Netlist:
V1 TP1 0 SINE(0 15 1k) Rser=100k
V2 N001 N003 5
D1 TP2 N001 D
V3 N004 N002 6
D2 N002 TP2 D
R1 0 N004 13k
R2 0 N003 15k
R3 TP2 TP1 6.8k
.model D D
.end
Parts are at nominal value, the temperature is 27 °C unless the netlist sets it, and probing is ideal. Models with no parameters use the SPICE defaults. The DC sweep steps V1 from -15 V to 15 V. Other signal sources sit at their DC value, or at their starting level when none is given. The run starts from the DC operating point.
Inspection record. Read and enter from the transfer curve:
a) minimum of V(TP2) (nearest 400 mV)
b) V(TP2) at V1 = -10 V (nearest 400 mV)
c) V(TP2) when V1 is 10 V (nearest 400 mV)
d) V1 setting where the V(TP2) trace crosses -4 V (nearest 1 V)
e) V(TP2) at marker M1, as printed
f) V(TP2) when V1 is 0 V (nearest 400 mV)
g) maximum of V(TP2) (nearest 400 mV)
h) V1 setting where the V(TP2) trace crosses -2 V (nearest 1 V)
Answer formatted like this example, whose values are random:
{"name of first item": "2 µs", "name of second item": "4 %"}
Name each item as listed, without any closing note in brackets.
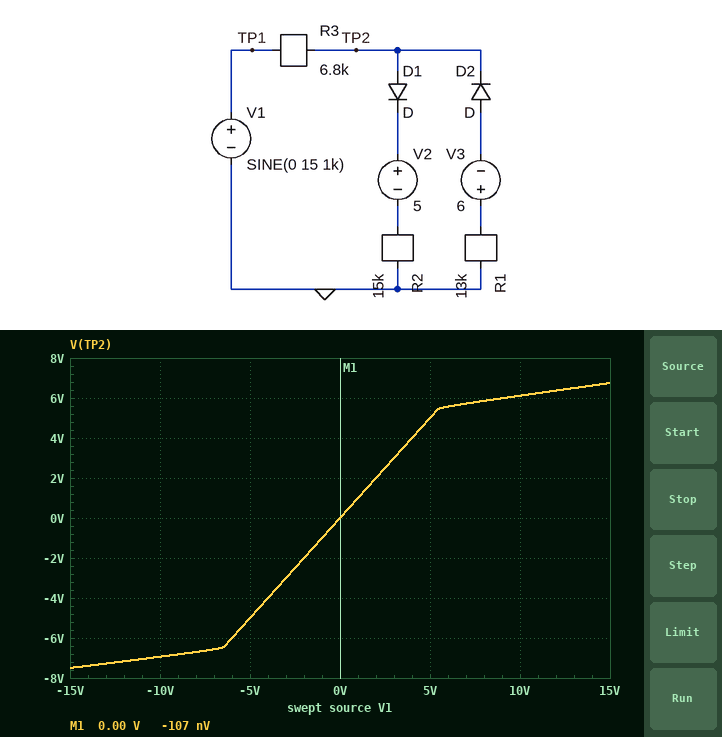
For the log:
{"minimum of V(TP2)": "-7.6 V", "V(TP2) at V1 = -10 V": "-6.8 V", "V(TP2) when V1 is 10 V": "6.0 V", "V1 setting where the V(TP2) trace crosses -4 V": "-4 V", "V(TP2) at marker M1, as printed": "-107 nV", "V(TP2) when V1 is 0 V": "0 V", "maximum of V(TP2)": "6.8 V", "V1 setting where the V(TP2) trace crosses -2 V": "-2 V"}
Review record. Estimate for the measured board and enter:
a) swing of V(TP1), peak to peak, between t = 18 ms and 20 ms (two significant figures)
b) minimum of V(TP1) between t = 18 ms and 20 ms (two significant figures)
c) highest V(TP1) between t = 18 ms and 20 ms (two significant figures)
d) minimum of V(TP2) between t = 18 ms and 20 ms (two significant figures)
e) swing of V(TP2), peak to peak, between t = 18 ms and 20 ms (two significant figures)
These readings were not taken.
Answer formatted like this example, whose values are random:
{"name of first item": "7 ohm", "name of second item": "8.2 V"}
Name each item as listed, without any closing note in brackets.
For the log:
{"swing of V(TP1), peak to peak, between t = 18 ms and 20 ms": "15 V", "minimum of V(TP1) between t = 18 ms and 20 ms": "-8.0 V", "highest V(TP1) between t = 18 ms and 20 ms": "7.3 V", "minimum of V(TP2) between t = 18 ms and 20 ms": "-7.5 V", "swing of V(TP2), peak to peak, between t = 18 ms and 20 ms": "14 V"}
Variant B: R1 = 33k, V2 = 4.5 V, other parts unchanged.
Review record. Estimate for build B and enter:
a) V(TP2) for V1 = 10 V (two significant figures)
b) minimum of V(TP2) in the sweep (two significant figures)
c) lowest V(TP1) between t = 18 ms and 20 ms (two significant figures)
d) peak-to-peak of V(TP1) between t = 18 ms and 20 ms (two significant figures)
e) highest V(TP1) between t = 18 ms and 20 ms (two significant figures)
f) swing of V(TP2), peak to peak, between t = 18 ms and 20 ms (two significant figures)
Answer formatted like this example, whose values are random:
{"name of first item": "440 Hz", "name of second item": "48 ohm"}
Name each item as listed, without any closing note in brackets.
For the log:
{"V(TP2) for V1 = 10 V": "5.7 V", "minimum of V(TP2) in the sweep": "-8.6 V", "lowest V(TP1) between t = 18 ms and 20 ms": "-9.0 V", "peak-to-peak of V(TP1) between t = 18 ms and 20 ms": "16 V", "highest V(TP1) between t = 18 ms and 20 ms": "6.9 V", "swing of V(TP2), peak to peak, between t = 18 ms and 20 ms": "15 V"}
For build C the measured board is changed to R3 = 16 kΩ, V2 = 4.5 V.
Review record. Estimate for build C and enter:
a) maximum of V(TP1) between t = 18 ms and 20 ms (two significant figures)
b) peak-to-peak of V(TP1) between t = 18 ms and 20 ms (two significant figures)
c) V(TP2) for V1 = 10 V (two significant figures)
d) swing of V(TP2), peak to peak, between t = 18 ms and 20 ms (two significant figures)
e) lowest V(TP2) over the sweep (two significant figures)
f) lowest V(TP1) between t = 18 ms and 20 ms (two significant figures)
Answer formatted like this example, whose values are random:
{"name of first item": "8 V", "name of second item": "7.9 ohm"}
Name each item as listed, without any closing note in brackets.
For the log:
{"maximum of V(TP1) between t = 18 ms and 20 ms": "7.4 V", "peak-to-peak of V(TP1) between t = 18 ms and 20 ms": "16 V", "V(TP2) for V1 = 10 V": "5.6 V", "swing of V(TP2), peak to peak, between t = 18 ms and 20 ms": "14 V", "lowest V(TP2) over the sweep": "-7.4 V", "lowest V(TP1) between t = 18 ms and 20 ms": "-8.5 V"}
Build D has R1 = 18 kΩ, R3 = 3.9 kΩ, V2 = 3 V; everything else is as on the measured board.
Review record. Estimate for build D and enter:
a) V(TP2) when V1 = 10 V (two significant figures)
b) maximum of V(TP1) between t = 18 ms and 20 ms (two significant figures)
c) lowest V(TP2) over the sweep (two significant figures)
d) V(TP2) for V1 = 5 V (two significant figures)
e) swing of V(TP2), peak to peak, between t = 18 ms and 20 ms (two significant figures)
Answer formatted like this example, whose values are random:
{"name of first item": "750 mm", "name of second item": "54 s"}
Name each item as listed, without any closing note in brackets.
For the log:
{"V(TP2) when V1 = 10 V": "4.4 V", "maximum of V(TP1) between t = 18 ms and 20 ms": "5.4 V", "lowest V(TP2) over the sweep": "-7.8 V", "V(TP2) for V1 = 5 V": "3.7 V", "swing of V(TP2), peak to peak, between t = 18 ms and 20 ms": "13 V"}
